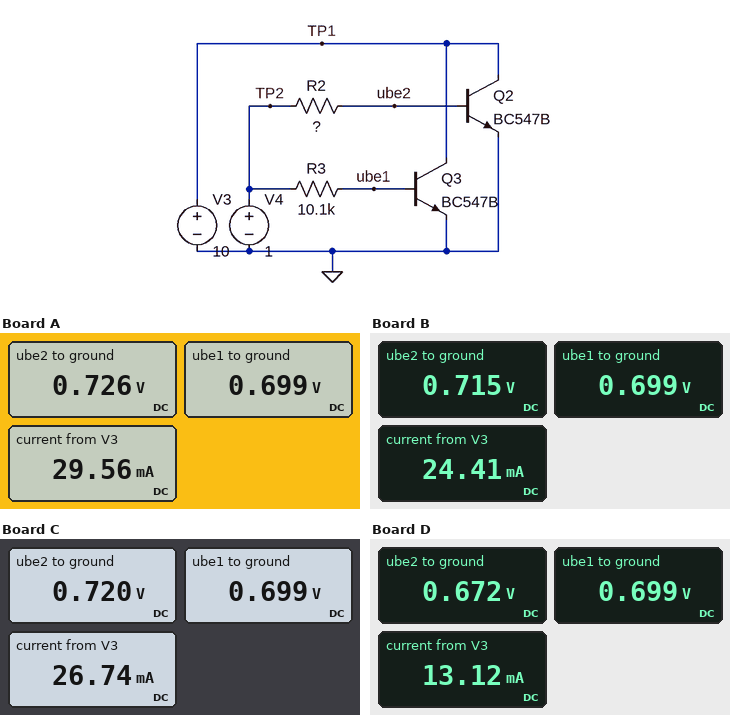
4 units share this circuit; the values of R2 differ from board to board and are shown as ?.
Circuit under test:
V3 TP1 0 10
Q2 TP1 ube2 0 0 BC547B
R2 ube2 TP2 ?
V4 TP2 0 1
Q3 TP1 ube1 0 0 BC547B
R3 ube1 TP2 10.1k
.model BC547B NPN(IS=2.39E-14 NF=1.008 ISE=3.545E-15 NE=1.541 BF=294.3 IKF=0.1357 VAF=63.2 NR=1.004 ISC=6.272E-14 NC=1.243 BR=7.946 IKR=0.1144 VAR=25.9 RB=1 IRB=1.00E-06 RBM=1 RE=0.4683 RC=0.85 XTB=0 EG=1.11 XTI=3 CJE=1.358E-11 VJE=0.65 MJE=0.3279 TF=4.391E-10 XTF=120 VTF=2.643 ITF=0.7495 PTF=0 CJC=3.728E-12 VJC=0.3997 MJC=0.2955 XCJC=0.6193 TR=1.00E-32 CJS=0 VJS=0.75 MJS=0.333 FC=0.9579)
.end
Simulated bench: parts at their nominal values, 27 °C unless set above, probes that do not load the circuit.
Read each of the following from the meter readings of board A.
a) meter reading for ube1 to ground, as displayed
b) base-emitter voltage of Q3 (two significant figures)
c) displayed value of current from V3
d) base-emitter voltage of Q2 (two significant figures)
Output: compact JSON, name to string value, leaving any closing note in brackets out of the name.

{"meter reading for ube1 to ground, as displayed": "0.699 V", "base-emitter voltage of Q3": "700 mV", "displayed value of current from V3": "29.56 mA", "base-emitter voltage of Q2": "730 mV"}
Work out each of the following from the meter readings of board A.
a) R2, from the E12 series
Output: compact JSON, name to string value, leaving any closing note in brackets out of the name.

{"R2, from the E12 series": "3.9 kΩ"}
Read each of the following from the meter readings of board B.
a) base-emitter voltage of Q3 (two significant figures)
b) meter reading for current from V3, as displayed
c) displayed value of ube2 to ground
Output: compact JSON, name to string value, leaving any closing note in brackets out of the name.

{"base-emitter voltage of Q3": "700 mV", "meter reading for current from V3, as displayed": "24.41 mA", "displayed value of ube2 to ground": "0.715 V"}
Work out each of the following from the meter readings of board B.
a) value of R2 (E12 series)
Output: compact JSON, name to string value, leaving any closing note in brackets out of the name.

{"value of R2": "5.6 kΩ"}
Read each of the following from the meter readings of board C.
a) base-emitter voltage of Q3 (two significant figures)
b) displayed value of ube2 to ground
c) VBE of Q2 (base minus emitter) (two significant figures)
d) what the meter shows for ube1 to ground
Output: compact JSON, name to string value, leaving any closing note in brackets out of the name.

{"base-emitter voltage of Q3": "700 mV", "displayed value of ube2 to ground": "0.720 V", "VBE of Q2 (base minus emitter)": "720 mV", "what the meter shows for ube1 to ground": "0.699 V"}
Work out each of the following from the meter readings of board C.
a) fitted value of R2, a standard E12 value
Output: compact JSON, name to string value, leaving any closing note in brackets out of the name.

{"fitted value of R2, a standard E12 value": "4.7 kΩ"}
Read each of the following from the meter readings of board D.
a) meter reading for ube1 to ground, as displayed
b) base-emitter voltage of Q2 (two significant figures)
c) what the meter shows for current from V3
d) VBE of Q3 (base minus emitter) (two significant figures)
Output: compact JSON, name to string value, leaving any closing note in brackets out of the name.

{"meter reading for ube1 to ground, as displayed": "0.699 V", "base-emitter voltage of Q2": "670 mV", "what the meter shows for current from V3": "13.12 mA", "VBE of Q3 (base minus emitter)": "700 mV"}
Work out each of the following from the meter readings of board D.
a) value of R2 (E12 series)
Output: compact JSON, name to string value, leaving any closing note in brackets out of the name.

{"value of R2": "27 kΩ"}
